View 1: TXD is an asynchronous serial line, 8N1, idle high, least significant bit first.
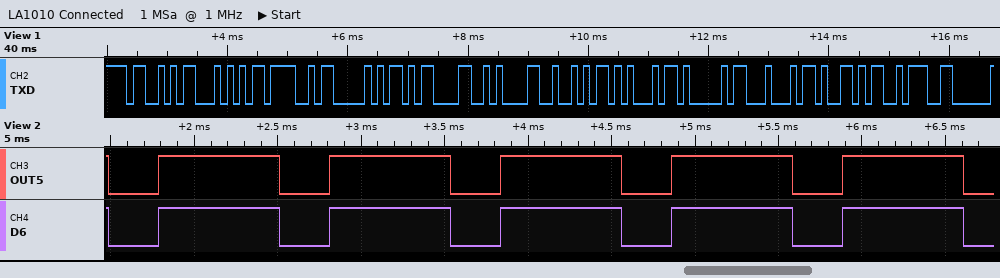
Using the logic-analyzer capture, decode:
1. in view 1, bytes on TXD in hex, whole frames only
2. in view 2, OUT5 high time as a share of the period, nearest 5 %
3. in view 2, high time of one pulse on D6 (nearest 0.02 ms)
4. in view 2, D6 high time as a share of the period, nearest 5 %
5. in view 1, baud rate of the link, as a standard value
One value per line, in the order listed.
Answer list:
53 54 4F 50 0D 0A 52 45 41 44 59 3A
70 %
0.72 ms
70 %
9600 baud
